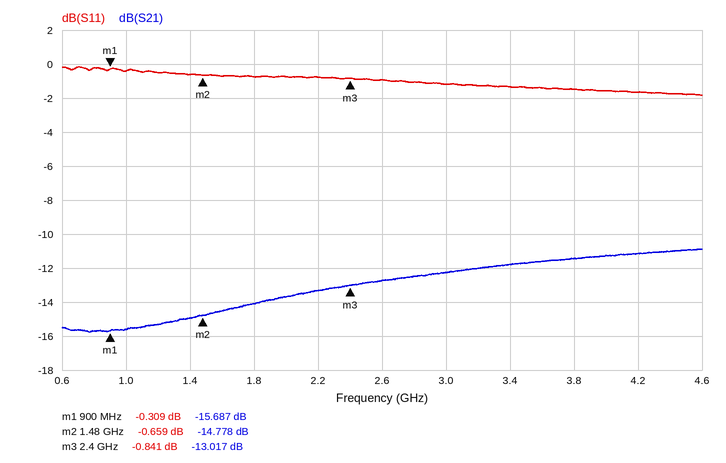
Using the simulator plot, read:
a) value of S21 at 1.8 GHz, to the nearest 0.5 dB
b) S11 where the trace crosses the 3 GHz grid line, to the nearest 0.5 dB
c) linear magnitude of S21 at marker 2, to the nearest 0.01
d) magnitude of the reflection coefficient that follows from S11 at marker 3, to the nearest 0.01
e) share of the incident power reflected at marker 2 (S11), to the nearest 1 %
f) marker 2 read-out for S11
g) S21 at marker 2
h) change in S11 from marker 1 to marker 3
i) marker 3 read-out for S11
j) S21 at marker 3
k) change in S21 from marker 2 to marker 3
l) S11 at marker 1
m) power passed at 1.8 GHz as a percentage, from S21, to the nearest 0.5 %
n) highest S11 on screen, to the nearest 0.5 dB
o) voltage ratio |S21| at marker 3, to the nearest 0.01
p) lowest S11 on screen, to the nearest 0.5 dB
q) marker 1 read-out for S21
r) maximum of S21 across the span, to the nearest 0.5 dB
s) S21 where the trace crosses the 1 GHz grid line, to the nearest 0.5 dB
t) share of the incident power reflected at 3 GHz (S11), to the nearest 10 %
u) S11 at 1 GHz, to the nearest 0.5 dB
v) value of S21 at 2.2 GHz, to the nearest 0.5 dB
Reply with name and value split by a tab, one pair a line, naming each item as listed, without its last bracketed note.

value of S21 at 1.8 GHz, to the nearest 0.5 dB	-14.0 dB
S11 where the trace crosses the 3 GHz grid line, to the nearest 0.5 dB	-1.0 dB
linear magnitude of S21 at marker 2, to the nearest 0.01	0.18
magnitude of the reflection coefficient that follows from S11 at marker 3, to the nearest 0.01	0.91
share of the incident power reflected at marker 2 (S11), to the nearest 1 %	86 %
marker 2 read-out for S11	-0.659 dB
S21 at marker 2	-14.778 dB
change in S11 from marker 1 to marker 3	-0.532 dB
marker 3 read-out for S11	-0.841 dB
S21 at marker 3	-13.017 dB
change in S21 from marker 2 to marker 3	1.761 dB
S11 at marker 1	-0.309 dB
power passed at 1.8 GHz as a percentage, from S21, to the nearest 0.5 %	4.0 %
highest S11 on screen, to the nearest 0.5 dB	0.0 dB
voltage ratio |S21| at marker 3, to the nearest 0.01	0.22
lowest S11 on screen, to the nearest 0.5 dB	-2.0 dB
marker 1 read-out for S21	-15.687 dB
maximum of S21 across the span, to the nearest 0.5 dB	-11.0 dB
S21 where the trace crosses the 1 GHz grid line, to the nearest 0.5 dB	-15.5 dB
share of the incident power reflected at 3 GHz (S11), to the nearest 10 %	80 %
S11 at 1 GHz, to the nearest 0.5 dB	-0.5 dB
value of S21 at 2.2 GHz, to the nearest 0.5 dB	-13.5 dB
